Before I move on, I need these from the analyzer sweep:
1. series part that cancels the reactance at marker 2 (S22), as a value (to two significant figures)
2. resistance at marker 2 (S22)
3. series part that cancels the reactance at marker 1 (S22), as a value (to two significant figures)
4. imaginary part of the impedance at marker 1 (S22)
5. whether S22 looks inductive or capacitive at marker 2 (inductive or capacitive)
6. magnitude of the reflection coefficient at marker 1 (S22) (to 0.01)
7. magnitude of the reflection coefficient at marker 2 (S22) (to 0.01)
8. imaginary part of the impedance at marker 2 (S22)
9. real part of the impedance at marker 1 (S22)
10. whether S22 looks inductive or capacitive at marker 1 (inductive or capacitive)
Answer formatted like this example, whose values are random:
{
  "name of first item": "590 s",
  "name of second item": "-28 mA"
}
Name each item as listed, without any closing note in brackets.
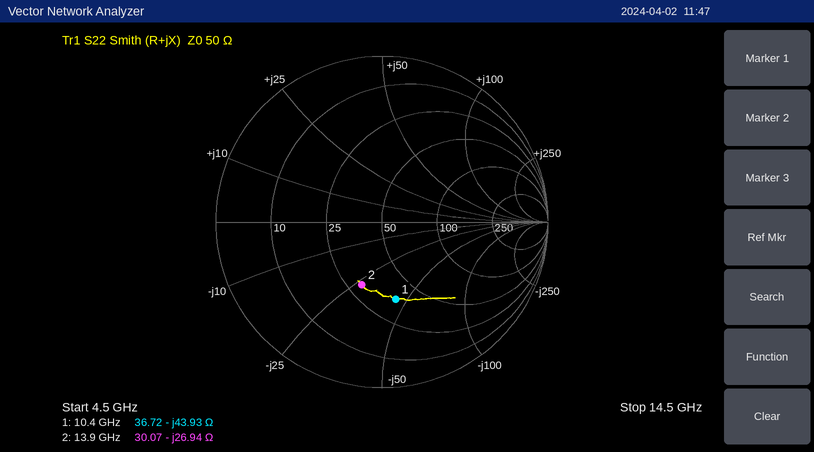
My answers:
{
  "series part that cancels the reactance at marker 2 (S22), as a value": "310 pH",
  "resistance at marker 2": "30.07 Ω",
  "series part that cancels the reactance at marker 1 (S22), as a value": "670 pH",
  "imaginary part of the impedance at marker 1": "-43.93 Ω",
  "whether S22 looks inductive or capacitive at marker 2": "capacitive",
  "magnitude of the reflection coefficient at marker 1 (S22)": "0.47",
  "magnitude of the reflection coefficient at marker 2 (S22)": "0.40",
  "imaginary part of the impedance at marker 2": "-26.94 Ω",
  "real part of the impedance at marker 1": "36.72 Ω",
  "whether S22 looks inductive or capacitive at marker 1": "capacitive"
}
